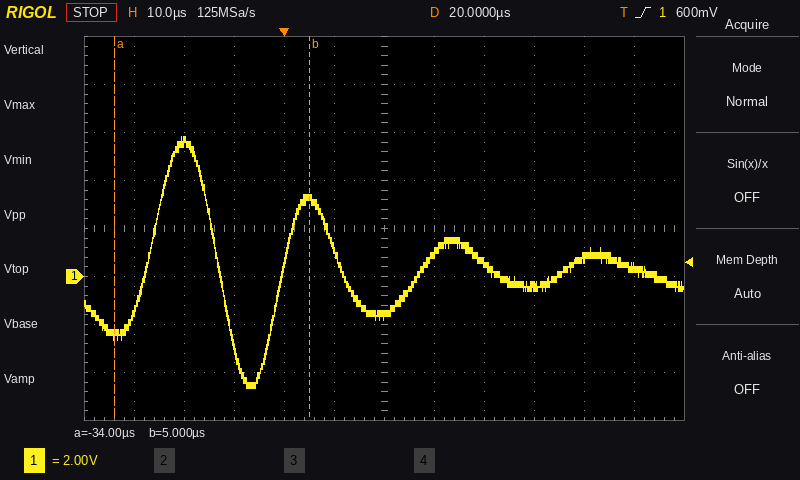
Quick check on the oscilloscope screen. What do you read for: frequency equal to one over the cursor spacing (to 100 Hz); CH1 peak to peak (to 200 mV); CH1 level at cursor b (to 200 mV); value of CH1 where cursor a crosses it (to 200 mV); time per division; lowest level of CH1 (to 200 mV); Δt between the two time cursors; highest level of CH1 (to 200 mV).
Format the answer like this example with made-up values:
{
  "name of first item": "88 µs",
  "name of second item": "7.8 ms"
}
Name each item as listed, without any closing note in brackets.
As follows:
{
  "frequency equal to one over the cursor spacing": "25.6 kHz",
  "CH1 peak to peak": "10.4 V",
  "CH1 level at cursor b": "3.2 V",
  "value of CH1 where cursor a crosses it": "-2.4 V",
  "time per division": "10 µs",
  "lowest level of CH1": "-4.6 V",
  "Δt between the two time cursors": "39 µs",
  "highest level of CH1": "5.8 V"
}
